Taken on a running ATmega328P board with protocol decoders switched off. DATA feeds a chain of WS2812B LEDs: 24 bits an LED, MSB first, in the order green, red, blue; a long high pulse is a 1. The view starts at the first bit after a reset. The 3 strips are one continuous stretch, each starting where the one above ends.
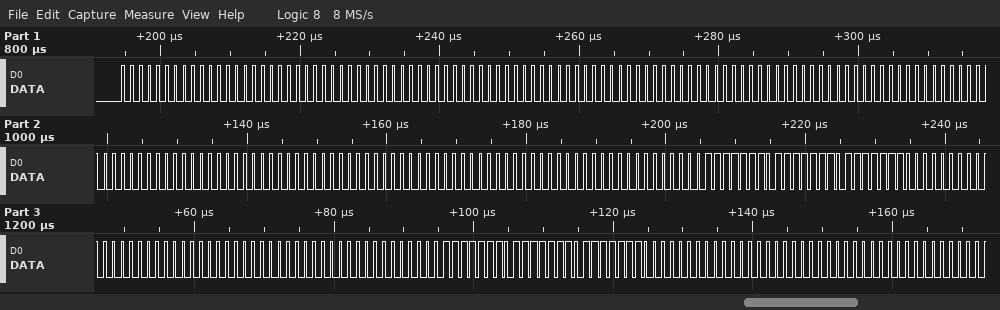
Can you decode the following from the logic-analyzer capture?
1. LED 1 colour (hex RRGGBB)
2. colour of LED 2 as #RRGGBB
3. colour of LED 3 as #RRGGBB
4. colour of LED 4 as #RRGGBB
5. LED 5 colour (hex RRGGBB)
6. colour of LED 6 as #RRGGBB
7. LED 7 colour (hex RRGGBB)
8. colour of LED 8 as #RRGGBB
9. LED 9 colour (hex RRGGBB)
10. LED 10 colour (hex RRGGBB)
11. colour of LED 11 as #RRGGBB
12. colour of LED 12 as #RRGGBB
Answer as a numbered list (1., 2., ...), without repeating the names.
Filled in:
1. #000000
2. #000000
3. #000000
4. #000000
5. #000000
6. #000000
7. #000000
8. #7F7F7F
9. #000000
10. #000000
11. #7F7F7F
12. #000000
